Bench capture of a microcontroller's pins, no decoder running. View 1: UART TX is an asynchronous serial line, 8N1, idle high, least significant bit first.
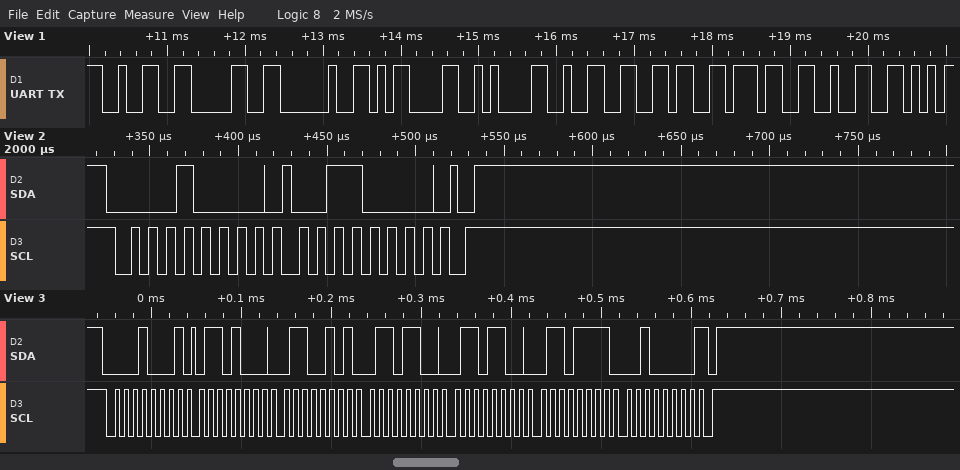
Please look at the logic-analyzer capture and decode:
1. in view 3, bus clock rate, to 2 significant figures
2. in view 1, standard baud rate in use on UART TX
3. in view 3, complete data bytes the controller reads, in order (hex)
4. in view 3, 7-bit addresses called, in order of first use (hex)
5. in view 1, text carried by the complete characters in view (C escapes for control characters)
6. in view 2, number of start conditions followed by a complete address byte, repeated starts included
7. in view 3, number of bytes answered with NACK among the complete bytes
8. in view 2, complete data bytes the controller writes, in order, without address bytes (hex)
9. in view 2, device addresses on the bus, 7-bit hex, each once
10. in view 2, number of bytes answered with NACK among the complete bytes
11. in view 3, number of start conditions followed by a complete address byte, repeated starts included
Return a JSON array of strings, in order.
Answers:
["100 kHz", "9600 baud", "68 65 6C 6C 6F 20", "0x08", "\"20 \\r\\n2672\"", "1", "1", "30", "0x08", "0", "1"]
